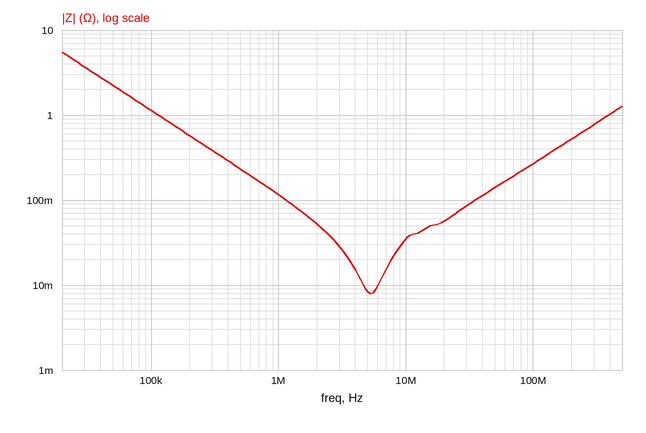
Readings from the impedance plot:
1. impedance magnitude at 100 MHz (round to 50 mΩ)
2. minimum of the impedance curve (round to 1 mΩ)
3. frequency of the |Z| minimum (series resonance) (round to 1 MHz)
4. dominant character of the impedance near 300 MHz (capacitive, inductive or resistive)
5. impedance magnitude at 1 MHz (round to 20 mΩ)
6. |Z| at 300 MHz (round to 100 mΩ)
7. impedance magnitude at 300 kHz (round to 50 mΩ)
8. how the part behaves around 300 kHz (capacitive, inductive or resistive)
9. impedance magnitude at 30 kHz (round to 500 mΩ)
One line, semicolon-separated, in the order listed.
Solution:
250 mΩ; 8 mΩ; 5 MHz; inductive; 120 mΩ; 800 mΩ; 400 mΩ; capacitive; 3.5 Ω
